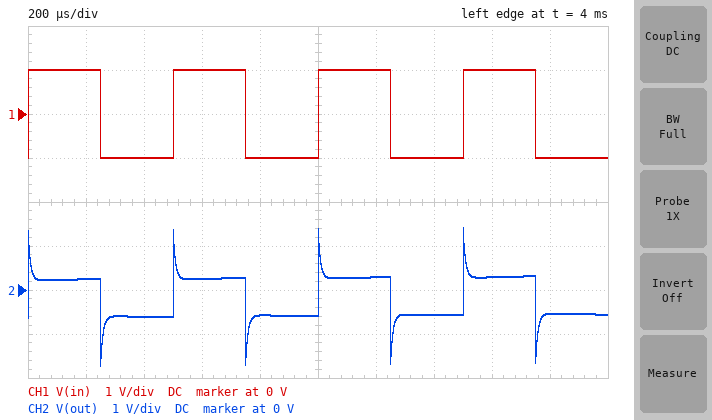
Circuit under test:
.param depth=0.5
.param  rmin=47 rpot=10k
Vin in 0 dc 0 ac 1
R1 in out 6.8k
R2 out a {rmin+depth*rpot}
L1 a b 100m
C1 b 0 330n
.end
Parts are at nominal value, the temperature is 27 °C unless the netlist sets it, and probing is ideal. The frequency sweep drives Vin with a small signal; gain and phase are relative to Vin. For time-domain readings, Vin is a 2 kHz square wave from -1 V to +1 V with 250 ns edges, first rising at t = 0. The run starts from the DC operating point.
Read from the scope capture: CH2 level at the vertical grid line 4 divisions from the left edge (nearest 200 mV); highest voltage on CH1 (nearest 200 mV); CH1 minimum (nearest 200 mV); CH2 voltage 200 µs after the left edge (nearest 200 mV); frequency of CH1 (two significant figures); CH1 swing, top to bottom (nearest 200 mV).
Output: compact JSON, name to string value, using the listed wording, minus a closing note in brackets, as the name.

{"CH2 level at the vertical grid line 4 divisions from the left edge": "-600 mV", "highest voltage on CH1": "1.0 V", "CH1 minimum": "-1.0 V", "CH2 voltage 200 µs after the left edge": "200 mV", "frequency of CH1": "2.0 kHz", "CH1 swing, top to bottom": "2.0 V"}
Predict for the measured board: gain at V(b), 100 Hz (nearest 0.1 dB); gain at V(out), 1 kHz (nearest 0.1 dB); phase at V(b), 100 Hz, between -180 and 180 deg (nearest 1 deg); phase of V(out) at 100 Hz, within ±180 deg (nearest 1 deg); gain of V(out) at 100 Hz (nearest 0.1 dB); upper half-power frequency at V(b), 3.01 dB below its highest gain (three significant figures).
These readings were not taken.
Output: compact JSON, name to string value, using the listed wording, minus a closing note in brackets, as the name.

{"gain at V(b), 100 Hz": "-8.5 dB", "gain at V(out), 1 kHz": "-7.4 dB", "phase at V(b), 100 Hz, between -180 and 180 deg": "-68 deg", "phase of V(out) at 100 Hz, within ±180 deg": "-21 deg", "gain of V(out) at 100 Hz": "-5.3 dB", "upper half-power frequency at V(b), 3.01 dB below its highest gain": "40.8 Hz"}
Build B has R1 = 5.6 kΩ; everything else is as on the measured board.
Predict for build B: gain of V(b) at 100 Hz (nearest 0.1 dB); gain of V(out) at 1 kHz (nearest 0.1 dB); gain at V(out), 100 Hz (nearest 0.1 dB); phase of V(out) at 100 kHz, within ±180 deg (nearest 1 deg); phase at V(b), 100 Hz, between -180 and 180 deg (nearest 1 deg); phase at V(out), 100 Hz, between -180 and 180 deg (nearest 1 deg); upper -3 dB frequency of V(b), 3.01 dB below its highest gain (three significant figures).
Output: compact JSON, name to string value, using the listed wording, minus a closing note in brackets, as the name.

{"gain of V(b) at 100 Hz": "-7.7 dB", "gain of V(out) at 1 kHz": "-6.5 dB", "gain at V(out), 100 Hz": "-4.5 dB", "phase of V(out) at 100 kHz, within ±180 deg": "5 deg", "phase at V(b), 100 Hz, between -180 and 180 deg": "-66 deg", "phase at V(out), 100 Hz, between -180 and 180 deg": "-19 deg", "upper -3 dB frequency of V(b), 3.01 dB below its highest gain": "45.4 Hz"}
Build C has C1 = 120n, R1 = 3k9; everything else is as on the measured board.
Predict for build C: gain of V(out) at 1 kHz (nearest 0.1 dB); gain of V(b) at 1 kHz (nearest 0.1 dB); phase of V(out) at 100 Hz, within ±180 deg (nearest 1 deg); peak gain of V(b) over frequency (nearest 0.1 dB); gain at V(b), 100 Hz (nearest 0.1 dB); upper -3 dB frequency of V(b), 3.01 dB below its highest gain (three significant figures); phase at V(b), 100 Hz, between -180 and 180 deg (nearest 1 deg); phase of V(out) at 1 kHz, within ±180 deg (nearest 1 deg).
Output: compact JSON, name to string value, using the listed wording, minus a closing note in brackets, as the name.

{"gain of V(out) at 1 kHz": "-4.9 dB", "gain of V(b) at 1 kHz": "-16.6 dB", "phase of V(out) at 100 Hz, within ±180 deg": "-13 deg", "peak gain of V(b) over frequency": "0 dB", "gain at V(b), 100 Hz": "-1.6 dB", "upper -3 dB frequency of V(b), 3.01 dB below its highest gain": "150 Hz", "phase at V(b), 100 Hz, between -180 and 180 deg": "-34 deg", "phase of V(out) at 1 kHz, within ±180 deg": "-3 deg"}
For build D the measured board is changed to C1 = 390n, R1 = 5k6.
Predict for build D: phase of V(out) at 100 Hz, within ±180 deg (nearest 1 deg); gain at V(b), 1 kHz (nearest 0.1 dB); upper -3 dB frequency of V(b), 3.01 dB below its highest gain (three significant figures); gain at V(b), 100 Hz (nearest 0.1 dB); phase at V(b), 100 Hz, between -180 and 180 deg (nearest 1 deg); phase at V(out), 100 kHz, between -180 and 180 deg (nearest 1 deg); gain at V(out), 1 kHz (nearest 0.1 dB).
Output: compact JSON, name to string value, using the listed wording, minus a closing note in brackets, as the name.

{"phase of V(out) at 100 Hz, within ±180 deg": "-18 deg", "gain at V(b), 1 kHz": "-28.3 dB", "upper -3 dB frequency of V(b), 3.01 dB below its highest gain": "38.4 Hz", "gain at V(b), 100 Hz": "-8.9 dB", "phase at V(b), 100 Hz, between -180 and 180 deg": "-69 deg", "phase at V(out), 100 kHz, between -180 and 180 deg": "5 deg", "gain at V(out), 1 kHz": "-6.5 dB"}
